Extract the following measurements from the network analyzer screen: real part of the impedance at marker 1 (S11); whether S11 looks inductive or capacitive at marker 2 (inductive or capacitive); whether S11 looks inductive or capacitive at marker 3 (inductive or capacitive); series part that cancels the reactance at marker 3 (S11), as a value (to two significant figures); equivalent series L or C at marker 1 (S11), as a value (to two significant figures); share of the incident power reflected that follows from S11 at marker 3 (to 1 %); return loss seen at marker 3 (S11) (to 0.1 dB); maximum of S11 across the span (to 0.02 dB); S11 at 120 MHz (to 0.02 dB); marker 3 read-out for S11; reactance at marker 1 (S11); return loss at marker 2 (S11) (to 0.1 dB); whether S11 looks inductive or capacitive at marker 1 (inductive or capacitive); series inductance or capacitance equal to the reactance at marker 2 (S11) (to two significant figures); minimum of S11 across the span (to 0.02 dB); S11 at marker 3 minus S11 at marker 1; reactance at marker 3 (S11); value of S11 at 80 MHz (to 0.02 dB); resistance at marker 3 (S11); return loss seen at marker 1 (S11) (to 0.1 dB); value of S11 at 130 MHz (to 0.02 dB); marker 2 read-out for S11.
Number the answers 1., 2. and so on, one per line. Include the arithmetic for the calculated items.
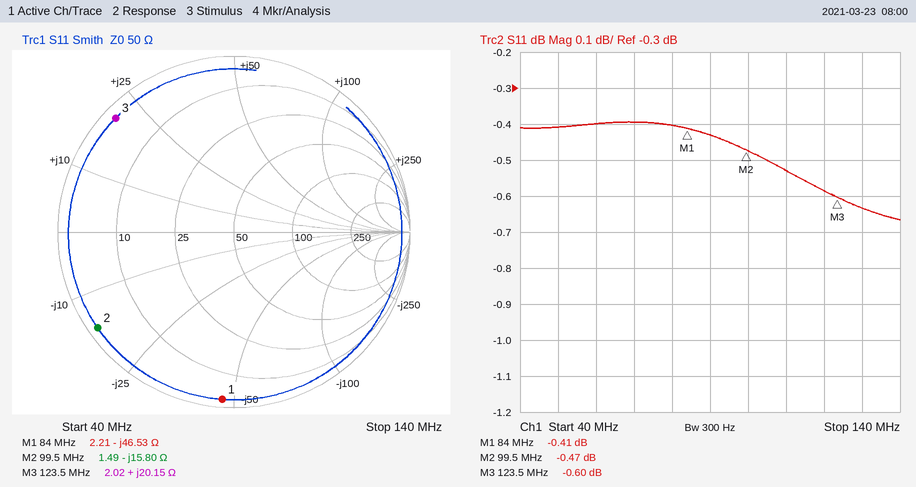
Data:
1. 2.21 Ω
2. capacitive
3. inductive
4. C = 1/(2π × 123.5 MHz × 20.15 Ω) ≈ 64 pF
5. C = 1/(2π × 84 MHz × 46.53 Ω) ≈ 41 pF
6. 10^(-0.6/10) ≈ 87 %
7. 0.6 dB
8. -0.40 dB
9. -0.58 dB
10. -0.60 dB
11. -46.53 Ω
12. 0.5 dB
13. capacitive
14. C = 1/(2π × 99.5 MHz × 15.8 Ω) ≈ 101 pF, so 100 pF to two significant figures
15. -0.66 dB
16. -0.6 − (-0.41) = -0.19 dB
17. +20.15 Ω
18. -0.40 dB
19. 2.02 Ω
20. 0.4 dB
21. -0.64 dB
22. -0.47 dB
